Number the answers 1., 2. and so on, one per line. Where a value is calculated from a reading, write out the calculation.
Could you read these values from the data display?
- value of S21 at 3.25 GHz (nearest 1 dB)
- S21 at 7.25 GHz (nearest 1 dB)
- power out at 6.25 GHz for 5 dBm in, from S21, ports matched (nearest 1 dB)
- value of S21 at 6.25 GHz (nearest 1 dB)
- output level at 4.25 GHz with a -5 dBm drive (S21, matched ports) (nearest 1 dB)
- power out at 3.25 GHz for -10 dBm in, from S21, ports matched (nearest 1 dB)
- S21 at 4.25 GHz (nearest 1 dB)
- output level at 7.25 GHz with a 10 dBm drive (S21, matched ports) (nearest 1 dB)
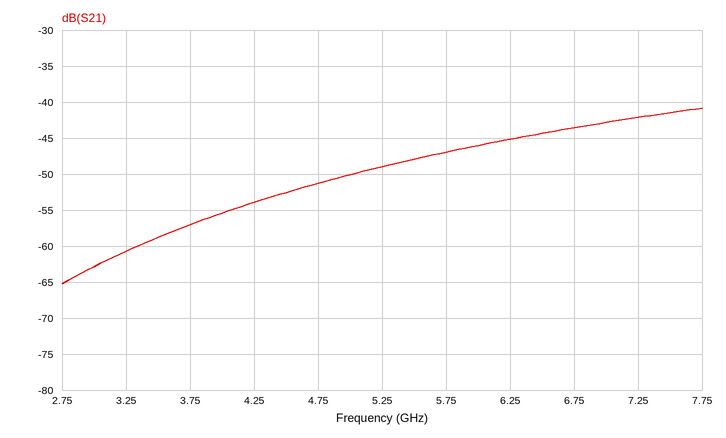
1. -61 dB
2. -42 dB
3. 5 dBm + (-45 dB) = -40 dBm
4. -45 dB
5. -5 dBm + (-54 dB) = -59 dBm
6. -10 dBm + (-61 dB) = -71 dBm
7. -54 dB
8. 10 dBm + (-42 dB) = -32 dBm
